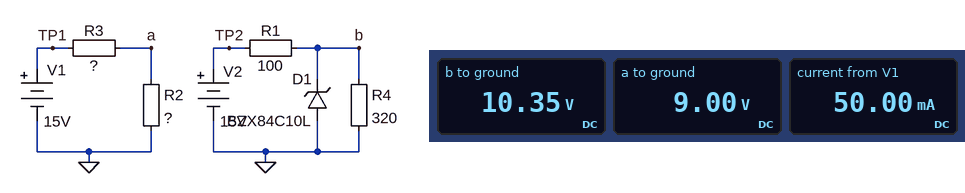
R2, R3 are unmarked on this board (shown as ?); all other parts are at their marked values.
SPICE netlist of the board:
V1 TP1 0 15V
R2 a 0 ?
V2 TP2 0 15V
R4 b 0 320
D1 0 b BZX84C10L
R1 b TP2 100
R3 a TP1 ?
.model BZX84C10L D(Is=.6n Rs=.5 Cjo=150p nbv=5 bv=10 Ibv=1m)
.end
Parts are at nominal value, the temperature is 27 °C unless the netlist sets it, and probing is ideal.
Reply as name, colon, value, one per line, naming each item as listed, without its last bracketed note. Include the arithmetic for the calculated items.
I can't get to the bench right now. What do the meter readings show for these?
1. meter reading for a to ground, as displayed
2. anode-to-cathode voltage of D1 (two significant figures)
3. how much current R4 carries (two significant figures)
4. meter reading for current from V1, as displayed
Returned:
meter reading for a to ground, as displayed: 9.00 V
anode-to-cathode voltage of D1: 0 V - 10.35 V = -10 V
how much current R4 carries: (10.35 V) / 320 Ω = 32 mA
meter reading for current from V1, as displayed: 50.00 mA
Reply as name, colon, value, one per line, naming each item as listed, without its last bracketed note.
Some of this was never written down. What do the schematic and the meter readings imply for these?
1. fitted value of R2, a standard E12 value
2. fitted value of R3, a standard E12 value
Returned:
fitted value of R2, a standard E12 value: 180 Ω
fitted value of R3, a standard E12 value: 120 Ω
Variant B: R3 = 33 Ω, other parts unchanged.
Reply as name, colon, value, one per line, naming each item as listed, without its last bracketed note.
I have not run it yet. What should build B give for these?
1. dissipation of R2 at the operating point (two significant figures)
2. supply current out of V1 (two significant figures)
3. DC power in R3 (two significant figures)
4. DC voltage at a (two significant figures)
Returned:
dissipation of R2 at the operating point: 890 mW
supply current out of V1: 70 mA
DC power in R3: 160 mW
DC voltage at a: 13 V
